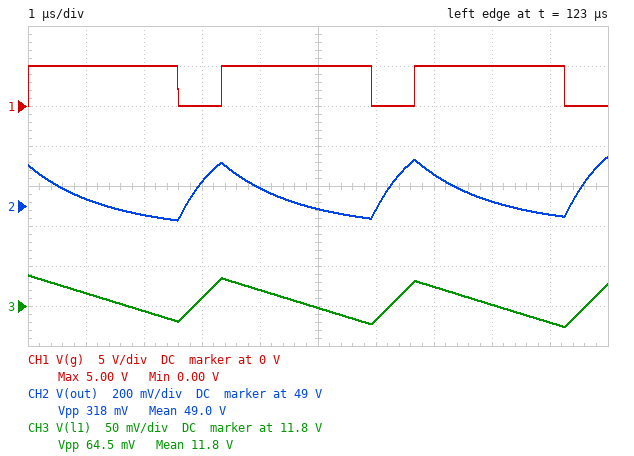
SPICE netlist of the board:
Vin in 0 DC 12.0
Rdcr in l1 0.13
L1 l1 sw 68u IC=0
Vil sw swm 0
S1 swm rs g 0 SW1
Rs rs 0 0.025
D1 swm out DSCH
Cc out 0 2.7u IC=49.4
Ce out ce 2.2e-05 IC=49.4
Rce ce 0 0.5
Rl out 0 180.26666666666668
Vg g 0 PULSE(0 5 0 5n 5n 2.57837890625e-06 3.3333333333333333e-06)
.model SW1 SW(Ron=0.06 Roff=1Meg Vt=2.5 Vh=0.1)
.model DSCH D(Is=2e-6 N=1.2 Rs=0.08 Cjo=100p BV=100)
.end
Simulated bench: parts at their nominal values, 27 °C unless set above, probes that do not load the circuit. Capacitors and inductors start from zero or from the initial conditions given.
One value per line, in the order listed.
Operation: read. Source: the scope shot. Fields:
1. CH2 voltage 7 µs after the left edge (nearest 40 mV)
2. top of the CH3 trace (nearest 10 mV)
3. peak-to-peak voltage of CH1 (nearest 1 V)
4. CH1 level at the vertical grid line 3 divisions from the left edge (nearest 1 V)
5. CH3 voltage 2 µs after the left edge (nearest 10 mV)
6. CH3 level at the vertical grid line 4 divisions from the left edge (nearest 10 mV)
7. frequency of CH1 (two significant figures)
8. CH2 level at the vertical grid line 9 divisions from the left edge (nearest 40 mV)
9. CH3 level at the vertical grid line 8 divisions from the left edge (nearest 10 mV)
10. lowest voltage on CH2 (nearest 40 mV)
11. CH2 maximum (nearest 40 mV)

49.16 V
11.84 V
5 V
0 V
11.79 V
11.82 V
300 kHz
48.96 V
11.80 V
48.92 V
49.24 V
